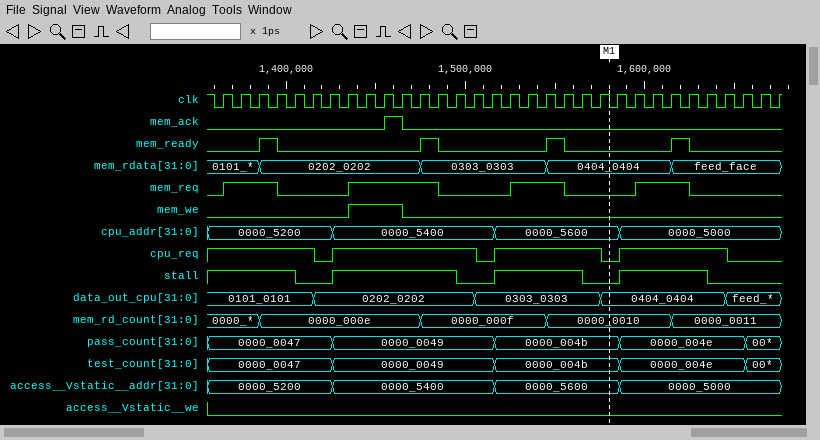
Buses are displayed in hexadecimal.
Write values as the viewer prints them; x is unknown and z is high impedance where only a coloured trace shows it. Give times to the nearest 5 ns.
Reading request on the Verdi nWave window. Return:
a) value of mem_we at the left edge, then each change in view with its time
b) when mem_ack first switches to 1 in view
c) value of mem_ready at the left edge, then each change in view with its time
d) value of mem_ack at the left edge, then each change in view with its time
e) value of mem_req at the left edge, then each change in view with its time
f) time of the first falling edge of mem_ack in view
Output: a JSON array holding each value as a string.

["0, 1 at 1435 ns, 0 at 1465 ns", "1455 ns", "0, 1 at 1385 ns, 0 at 1395 ns, 1 at 1475 ns, 0 at 1485 ns, 1 at 1545 ns, 0 at 1555 ns, 1 at 1615 ns, 0 at 1625 ns", "0, 1 at 1455 ns, 0 at 1465 ns", "0, 1 at 1365 ns, 0 at 1395 ns, 1 at 1435 ns, 0 at 1485 ns, 1 at 1525 ns, 0 at 1555 ns, 1 at 1595 ns, 0 at 1625 ns", "1465 ns"]
